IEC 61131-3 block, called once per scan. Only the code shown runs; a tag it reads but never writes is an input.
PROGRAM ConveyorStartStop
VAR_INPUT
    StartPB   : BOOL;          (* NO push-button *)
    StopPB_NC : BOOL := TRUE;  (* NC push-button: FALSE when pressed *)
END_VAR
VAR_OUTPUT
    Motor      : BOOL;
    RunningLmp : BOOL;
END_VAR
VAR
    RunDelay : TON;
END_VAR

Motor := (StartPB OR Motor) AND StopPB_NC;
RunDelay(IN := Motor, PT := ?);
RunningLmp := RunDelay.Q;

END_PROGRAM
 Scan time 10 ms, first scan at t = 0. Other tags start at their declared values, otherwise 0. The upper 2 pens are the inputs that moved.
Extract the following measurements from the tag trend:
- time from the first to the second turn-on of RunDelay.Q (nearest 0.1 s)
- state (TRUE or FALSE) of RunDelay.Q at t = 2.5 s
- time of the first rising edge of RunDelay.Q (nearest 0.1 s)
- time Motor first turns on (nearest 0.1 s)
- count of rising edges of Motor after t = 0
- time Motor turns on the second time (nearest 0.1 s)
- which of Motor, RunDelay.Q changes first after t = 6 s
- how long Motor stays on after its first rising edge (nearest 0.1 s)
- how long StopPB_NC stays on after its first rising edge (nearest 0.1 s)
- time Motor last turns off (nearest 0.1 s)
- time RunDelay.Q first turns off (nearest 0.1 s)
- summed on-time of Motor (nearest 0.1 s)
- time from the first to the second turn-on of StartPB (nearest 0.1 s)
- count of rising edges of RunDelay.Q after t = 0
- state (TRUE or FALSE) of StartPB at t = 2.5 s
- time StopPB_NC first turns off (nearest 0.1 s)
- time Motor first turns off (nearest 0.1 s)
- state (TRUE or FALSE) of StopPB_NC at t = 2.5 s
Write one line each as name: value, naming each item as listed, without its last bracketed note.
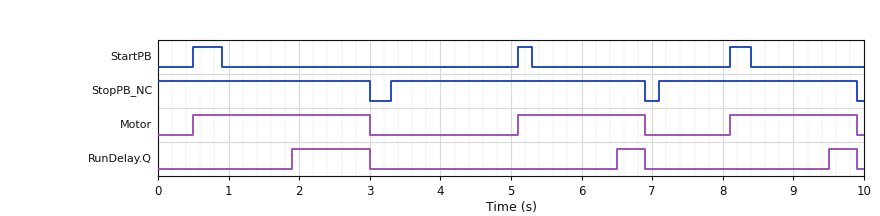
time from the first to the second turn-on of RunDelay.Q: 4.6 s
state (TRUE or FALSE) of RunDelay.Q at t = 2.5 s: TRUE
time of the first rising edge of RunDelay.Q: 1.9 s
time Motor first turns on: 0.5 s
count of rising edges of Motor after t = 0: 3
time Motor turns on the second time: 5.1 s
which of Motor, RunDelay.Q changes first after t = 6 s: RunDelay.Q
how long Motor stays on after its first rising edge: 2.5 s
how long StopPB_NC stays on after its first rising edge: 3.6 s
time Motor last turns off: 9.9 s
time RunDelay.Q first turns off: 3.0 s
summed on-time of Motor: 6.1 s
time from the first to the second turn-on of StartPB: 4.6 s
count of rising edges of RunDelay.Q after t = 0: 3
state (TRUE or FALSE) of StartPB at t = 2.5 s: FALSE
time StopPB_NC first turns off: 3.0 s
time Motor first turns off: 3.0 s
state (TRUE or FALSE) of StopPB_NC at t = 2.5 s: TRUE
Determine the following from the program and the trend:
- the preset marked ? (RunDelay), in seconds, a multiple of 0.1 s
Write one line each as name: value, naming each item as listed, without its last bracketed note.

the preset marked ? (RunDelay), in seconds, a multiple of 0.1 s: 1.4 s
